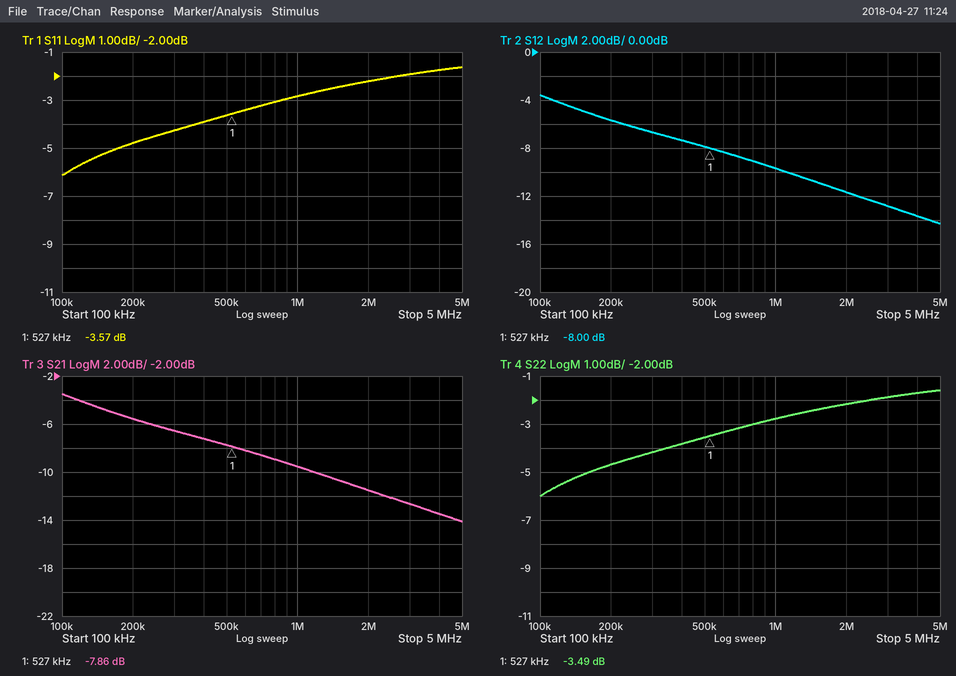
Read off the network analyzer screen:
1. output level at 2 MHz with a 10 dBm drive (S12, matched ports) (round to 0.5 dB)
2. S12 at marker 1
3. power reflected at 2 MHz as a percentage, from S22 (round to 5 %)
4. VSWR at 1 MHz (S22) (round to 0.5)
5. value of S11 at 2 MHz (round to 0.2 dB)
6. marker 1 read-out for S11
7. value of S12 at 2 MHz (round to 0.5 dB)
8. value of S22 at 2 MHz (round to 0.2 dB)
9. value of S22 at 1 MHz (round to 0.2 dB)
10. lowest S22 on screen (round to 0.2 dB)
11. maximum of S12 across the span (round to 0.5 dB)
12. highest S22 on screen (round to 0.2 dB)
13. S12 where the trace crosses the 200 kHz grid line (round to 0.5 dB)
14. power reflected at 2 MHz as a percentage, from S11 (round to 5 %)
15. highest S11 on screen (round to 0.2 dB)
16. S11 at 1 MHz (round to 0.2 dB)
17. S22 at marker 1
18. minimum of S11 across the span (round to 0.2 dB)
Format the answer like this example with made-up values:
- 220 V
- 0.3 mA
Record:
- -1.5 dBm
- -8.00 dB
- 60 %
- 6.5
- -2.2 dB
- -3.57 dB
- -11.5 dB
- -2.2 dB
- -2.8 dB
- -6.0 dB
- -3.5 dB
- -1.6 dB
- -5.5 dB
- 60 %
- -1.6 dB
- -2.8 dB
- -3.49 dB
- -6.2 dB
